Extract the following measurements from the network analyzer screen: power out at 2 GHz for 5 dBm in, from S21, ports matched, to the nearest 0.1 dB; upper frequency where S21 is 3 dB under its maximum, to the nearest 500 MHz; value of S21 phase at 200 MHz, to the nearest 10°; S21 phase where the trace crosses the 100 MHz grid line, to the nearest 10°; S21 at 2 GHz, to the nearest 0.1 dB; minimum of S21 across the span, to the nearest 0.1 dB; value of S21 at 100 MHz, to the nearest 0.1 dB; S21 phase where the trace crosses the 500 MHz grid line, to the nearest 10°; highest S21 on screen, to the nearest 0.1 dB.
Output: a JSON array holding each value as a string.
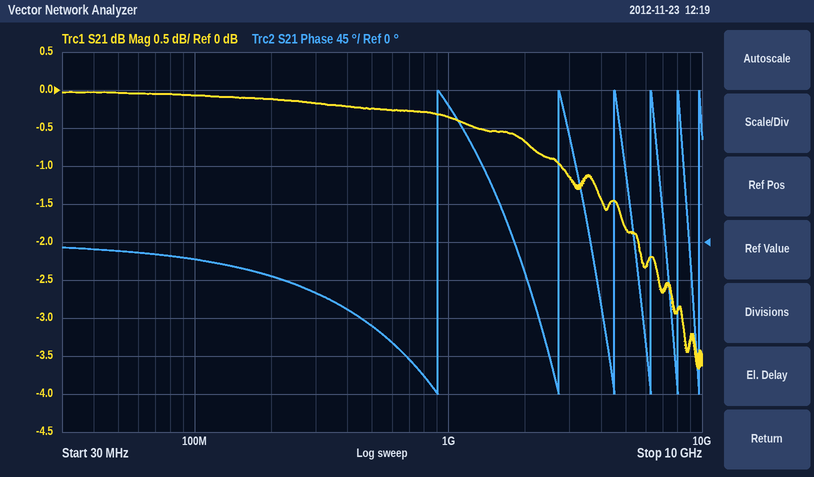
["4.3 dBm", "8.5 GHz", "-40°", "-20°", "-0.7 dB", "-3.7 dB", "-0.1 dB", "-100°", "0.0 dB"]
